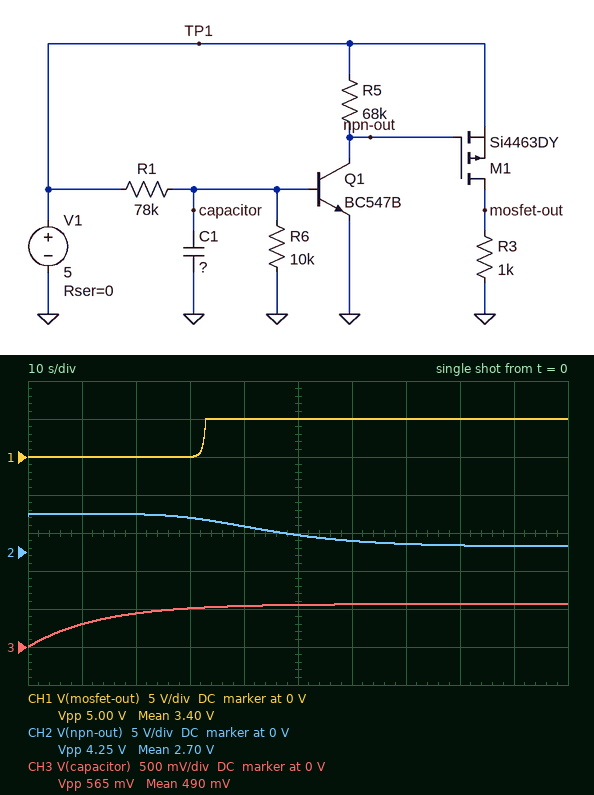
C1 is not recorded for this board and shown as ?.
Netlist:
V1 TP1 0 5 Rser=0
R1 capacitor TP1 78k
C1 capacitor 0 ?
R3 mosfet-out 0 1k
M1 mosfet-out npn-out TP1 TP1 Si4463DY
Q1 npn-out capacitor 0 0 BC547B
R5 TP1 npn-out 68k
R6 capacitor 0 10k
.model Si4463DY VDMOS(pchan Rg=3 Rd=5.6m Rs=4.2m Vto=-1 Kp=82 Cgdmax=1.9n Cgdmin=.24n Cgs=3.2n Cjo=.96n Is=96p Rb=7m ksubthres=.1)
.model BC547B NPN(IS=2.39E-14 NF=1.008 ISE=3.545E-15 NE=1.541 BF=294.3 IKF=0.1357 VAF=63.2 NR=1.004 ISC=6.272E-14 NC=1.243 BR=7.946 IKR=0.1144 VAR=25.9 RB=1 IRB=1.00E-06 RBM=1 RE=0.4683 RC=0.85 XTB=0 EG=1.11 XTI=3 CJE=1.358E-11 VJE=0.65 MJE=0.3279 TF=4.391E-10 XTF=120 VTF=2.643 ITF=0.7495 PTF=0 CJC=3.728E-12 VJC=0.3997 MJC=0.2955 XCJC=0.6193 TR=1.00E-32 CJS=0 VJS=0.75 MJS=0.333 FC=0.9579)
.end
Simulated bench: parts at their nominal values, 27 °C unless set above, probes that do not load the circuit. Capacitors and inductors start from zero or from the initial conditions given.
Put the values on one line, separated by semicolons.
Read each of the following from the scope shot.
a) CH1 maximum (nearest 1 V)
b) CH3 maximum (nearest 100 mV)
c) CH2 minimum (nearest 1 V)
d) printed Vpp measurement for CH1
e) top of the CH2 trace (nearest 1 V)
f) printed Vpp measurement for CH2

5 V; 600 mV; 1 V; 5.00 V; 5 V; 4.25 V
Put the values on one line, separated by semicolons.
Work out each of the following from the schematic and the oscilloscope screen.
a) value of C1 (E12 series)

1.5 mF
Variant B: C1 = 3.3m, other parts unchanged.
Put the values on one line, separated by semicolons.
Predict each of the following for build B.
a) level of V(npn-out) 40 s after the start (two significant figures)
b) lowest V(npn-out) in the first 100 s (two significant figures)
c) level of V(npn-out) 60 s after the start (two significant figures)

5.0 V; 2.7 V; 4.7 V
